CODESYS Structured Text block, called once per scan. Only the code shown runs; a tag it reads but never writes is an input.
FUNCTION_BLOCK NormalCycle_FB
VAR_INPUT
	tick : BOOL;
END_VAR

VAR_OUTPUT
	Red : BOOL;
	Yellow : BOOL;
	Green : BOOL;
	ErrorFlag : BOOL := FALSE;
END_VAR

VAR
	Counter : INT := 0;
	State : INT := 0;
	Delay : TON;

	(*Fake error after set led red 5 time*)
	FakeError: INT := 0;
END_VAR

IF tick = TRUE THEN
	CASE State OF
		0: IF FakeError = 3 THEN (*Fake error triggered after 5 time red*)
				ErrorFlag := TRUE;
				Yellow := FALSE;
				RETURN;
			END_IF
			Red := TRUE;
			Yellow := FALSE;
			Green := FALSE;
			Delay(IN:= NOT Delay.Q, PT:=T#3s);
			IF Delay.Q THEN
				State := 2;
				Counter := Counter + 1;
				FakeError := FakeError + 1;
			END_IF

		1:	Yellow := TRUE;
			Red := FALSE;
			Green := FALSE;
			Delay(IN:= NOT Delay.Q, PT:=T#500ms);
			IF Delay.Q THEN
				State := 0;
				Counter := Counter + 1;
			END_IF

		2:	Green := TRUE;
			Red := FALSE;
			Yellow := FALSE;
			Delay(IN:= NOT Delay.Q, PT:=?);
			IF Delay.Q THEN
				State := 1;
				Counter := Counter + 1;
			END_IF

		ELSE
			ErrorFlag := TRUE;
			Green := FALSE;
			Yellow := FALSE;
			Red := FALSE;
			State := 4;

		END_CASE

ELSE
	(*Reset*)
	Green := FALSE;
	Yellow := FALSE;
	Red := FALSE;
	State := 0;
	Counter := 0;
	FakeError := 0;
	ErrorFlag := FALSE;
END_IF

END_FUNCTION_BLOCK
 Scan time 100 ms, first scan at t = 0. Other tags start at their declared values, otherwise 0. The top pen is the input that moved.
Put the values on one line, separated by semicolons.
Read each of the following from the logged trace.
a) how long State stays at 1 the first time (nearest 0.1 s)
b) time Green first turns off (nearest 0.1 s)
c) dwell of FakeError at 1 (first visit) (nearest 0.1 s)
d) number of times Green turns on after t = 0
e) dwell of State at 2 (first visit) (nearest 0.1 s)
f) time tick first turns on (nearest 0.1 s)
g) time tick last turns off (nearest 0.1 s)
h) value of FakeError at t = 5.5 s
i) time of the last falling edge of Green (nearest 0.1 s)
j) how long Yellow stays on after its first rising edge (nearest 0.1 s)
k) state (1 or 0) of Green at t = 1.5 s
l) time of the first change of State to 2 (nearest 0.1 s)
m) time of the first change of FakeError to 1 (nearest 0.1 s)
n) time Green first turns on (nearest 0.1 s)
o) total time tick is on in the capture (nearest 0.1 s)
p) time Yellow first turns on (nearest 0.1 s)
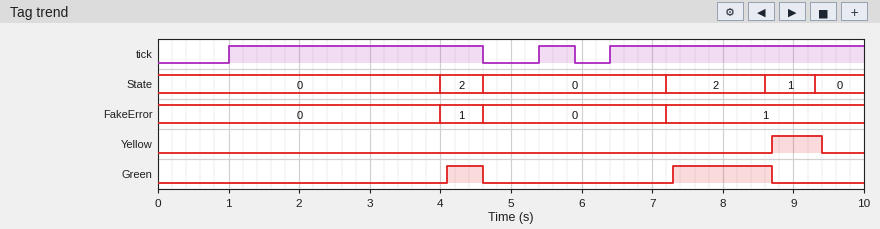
0.7 s; 4.6 s; 0.6 s; 2; 0.6 s; 1.0 s; 5.9 s; 0; 8.7 s; 0.7 s; 0; 4.0 s; 4.0 s; 4.1 s; 7.7 s; 8.7 s
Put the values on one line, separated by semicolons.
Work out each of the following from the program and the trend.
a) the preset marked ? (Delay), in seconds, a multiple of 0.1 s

1.2 s
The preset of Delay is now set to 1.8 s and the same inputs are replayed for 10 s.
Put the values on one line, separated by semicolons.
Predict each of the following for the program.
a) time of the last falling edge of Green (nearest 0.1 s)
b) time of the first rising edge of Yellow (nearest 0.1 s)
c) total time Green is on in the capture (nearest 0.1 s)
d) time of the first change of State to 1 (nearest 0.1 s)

9.3 s; 9.3 s; 2.5 s; 9.2 s
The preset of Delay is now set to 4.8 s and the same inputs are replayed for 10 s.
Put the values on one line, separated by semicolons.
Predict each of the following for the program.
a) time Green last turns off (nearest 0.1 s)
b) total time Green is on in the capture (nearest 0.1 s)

4.6 s; 3.2 s
